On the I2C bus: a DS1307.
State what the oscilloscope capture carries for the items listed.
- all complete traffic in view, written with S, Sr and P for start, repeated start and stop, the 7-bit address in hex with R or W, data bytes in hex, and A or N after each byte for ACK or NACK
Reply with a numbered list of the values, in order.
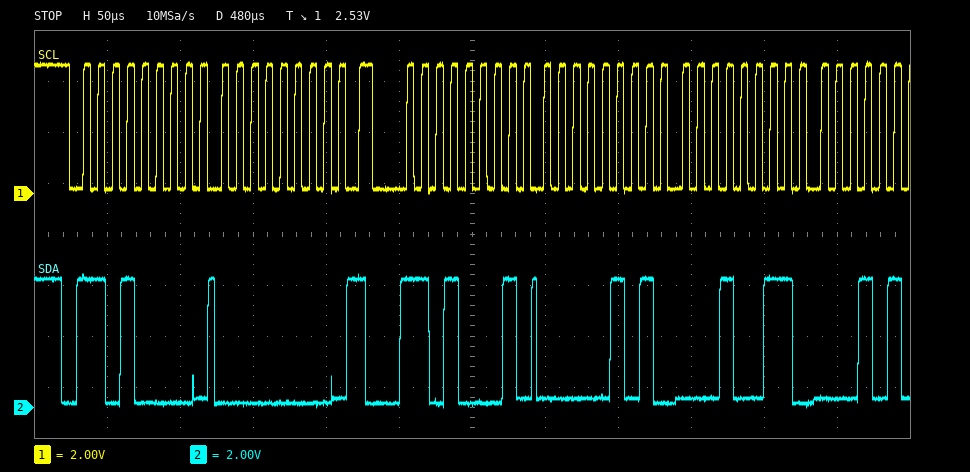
1. S 68W A 00 A Sr 68R A 05 A 13 A
